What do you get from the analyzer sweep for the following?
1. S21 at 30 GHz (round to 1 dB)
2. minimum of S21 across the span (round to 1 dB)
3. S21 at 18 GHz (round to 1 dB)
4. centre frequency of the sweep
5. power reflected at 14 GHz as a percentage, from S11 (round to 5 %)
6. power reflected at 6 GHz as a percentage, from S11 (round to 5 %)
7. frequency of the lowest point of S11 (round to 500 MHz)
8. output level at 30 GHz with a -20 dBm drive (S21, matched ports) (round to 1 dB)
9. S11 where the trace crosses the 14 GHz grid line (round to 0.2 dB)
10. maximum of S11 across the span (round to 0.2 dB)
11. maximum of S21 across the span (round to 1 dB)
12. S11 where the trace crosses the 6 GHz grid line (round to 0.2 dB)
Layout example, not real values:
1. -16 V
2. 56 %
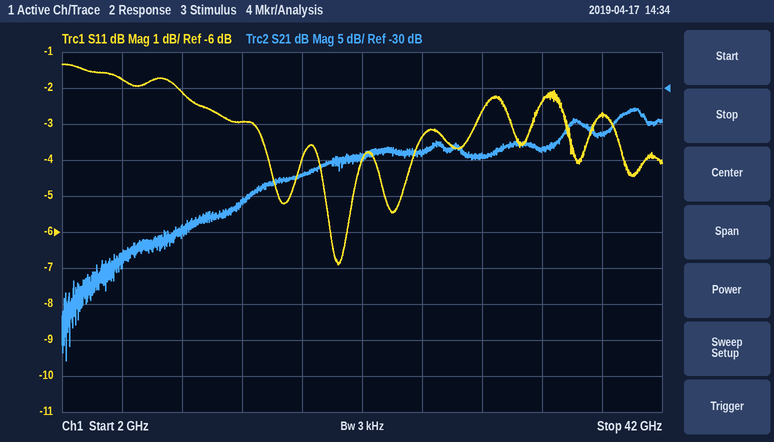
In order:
1. -39 dB
2. -68 dB
3. -42 dB
4. 22 GHz
5. 50 %
6. 65 %
7. 20.5 GHz
8. -59 dBm
9. -3.0 dB
10. -1.4 dB
11. -33 dB
12. -1.8 dB
